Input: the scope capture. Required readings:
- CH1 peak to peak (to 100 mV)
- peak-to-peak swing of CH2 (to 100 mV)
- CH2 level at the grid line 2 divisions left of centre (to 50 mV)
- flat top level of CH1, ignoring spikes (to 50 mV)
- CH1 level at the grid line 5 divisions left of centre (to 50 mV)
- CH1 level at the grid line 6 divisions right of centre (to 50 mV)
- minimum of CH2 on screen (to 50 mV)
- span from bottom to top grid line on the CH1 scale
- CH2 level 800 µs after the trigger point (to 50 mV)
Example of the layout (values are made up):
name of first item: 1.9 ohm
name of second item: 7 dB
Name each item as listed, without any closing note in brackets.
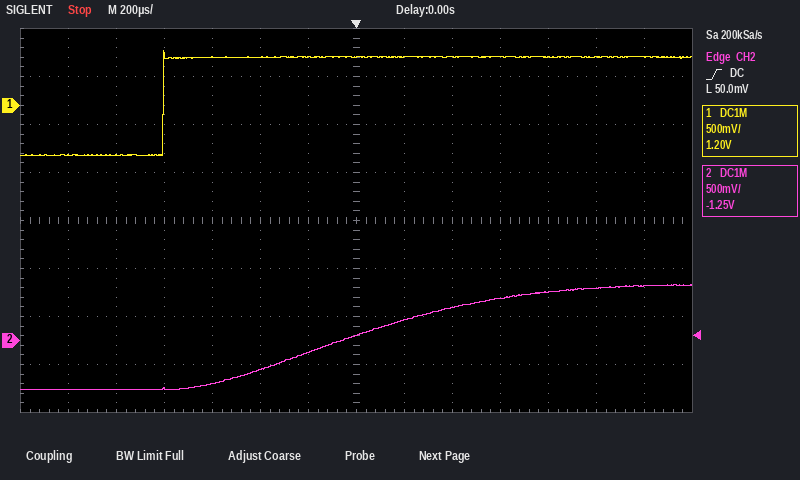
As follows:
CH1 peak to peak: 1.10 V
peak-to-peak swing of CH2: 1.10 V
CH2 level at the grid line 2 divisions left of centre: -300 mV
flat top level of CH1, ignoring spikes: 500 mV
CH1 level at the grid line 5 divisions left of centre: -500 mV
CH1 level at the grid line 6 divisions right of centre: 500 mV
minimum of CH2 on screen: -500 mV
span from bottom to top grid line on the CH1 scale: 4 V
CH2 level 800 µs after the trigger point: 500 mV
